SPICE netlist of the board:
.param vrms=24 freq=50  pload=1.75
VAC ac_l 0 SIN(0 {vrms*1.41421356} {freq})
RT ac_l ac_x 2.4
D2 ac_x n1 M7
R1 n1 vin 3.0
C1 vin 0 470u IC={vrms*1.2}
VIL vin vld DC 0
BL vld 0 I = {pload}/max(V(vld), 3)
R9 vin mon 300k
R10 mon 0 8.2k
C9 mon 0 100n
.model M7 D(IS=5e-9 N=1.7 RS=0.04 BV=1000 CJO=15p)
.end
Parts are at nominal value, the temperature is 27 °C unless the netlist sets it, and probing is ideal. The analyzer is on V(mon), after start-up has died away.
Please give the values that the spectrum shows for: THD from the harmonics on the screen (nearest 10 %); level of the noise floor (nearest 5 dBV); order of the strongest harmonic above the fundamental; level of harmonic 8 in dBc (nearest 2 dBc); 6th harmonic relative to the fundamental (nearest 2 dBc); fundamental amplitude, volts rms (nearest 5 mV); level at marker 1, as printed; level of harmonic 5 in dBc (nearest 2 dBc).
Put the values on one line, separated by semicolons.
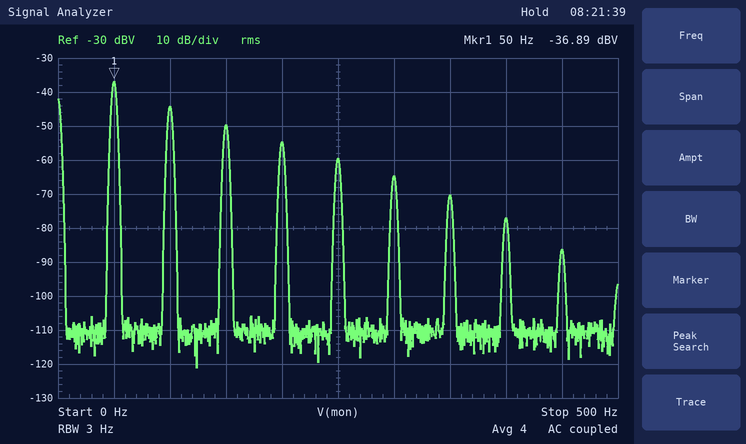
50 %; -110 dBV; 2; -40 dBc; -28 dBc; 15 mV; -36.89 dBV; -22 dBc
